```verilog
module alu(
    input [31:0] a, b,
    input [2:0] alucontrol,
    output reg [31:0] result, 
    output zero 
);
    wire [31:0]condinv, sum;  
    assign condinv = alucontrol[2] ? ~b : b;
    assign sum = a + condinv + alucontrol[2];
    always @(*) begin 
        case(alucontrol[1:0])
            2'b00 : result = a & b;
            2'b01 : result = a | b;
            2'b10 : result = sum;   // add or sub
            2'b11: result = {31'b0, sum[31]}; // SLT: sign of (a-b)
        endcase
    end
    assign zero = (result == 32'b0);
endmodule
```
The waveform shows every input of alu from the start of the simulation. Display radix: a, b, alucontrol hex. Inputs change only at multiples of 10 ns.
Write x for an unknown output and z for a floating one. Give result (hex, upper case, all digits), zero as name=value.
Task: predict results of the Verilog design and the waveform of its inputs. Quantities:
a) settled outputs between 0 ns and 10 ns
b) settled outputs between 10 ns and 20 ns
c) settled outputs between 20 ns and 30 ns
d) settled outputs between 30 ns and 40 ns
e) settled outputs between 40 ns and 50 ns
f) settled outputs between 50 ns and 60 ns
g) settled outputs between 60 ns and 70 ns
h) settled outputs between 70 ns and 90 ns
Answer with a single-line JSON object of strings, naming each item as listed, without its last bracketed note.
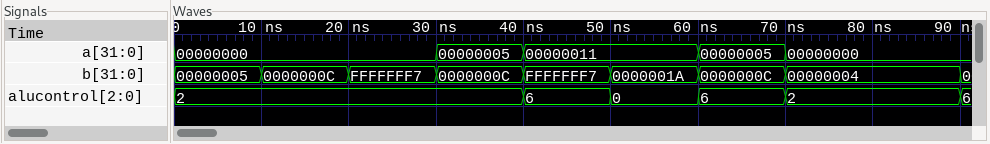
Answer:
{"settled outputs between 0 ns and 10 ns": "result=00000005, zero=0", "settled outputs between 10 ns and 20 ns": "result=0000000C, zero=0", "settled outputs between 20 ns and 30 ns": "result=FFFFFFF7, zero=0", "settled outputs between 30 ns and 40 ns": "result=00000011, zero=0", "settled outputs between 40 ns and 50 ns": "result=0000001A, zero=0", "settled outputs between 50 ns and 60 ns": "result=00000010, zero=0", "settled outputs between 60 ns and 70 ns": "result=FFFFFFF9, zero=0", "settled outputs between 70 ns and 90 ns": "result=00000004, zero=0"}
